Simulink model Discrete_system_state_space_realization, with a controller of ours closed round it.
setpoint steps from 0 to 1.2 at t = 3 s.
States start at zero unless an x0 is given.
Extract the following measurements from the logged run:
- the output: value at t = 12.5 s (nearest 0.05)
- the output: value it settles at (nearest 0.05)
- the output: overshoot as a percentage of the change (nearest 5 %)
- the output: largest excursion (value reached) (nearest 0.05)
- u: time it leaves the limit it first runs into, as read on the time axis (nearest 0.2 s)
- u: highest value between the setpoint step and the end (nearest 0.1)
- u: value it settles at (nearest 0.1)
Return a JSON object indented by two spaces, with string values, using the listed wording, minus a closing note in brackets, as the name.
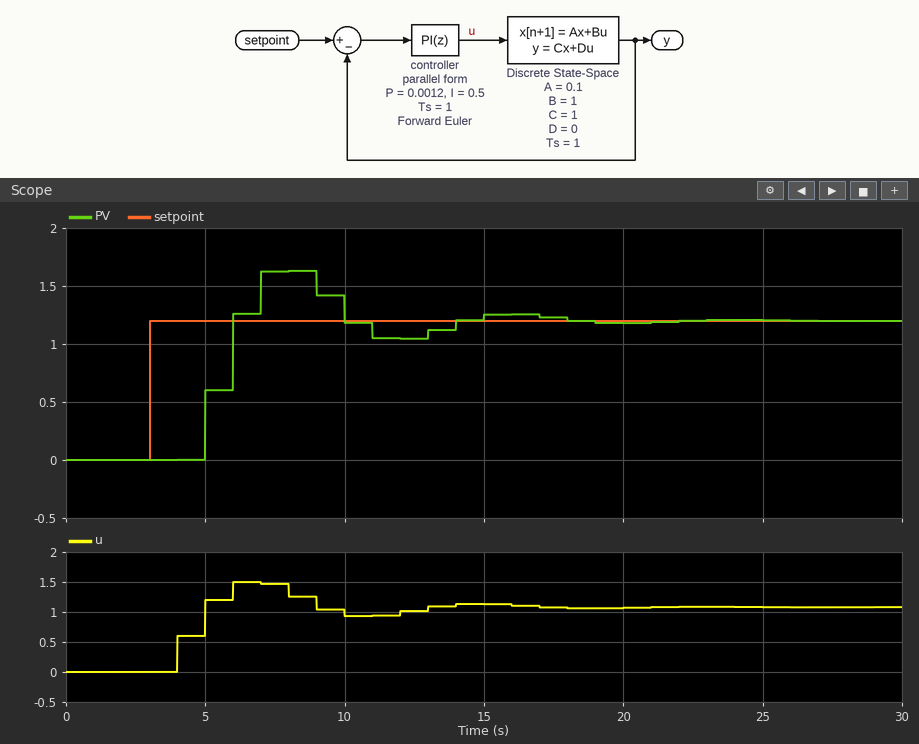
{
  "the output: value at t = 12.5 s": "1.05",
  "the output: value it settles at": "1.20",
  "the output: overshoot as a percentage of the change": "35 %",
  "the output: largest excursion (value reached)": "1.65",
  "u: time it leaves the limit it first runs into, as read on the time axis": "4.0 s",
  "u: highest value between the setpoint step and the end": "1.5",
  "u: value it settles at": "1.1"
}
